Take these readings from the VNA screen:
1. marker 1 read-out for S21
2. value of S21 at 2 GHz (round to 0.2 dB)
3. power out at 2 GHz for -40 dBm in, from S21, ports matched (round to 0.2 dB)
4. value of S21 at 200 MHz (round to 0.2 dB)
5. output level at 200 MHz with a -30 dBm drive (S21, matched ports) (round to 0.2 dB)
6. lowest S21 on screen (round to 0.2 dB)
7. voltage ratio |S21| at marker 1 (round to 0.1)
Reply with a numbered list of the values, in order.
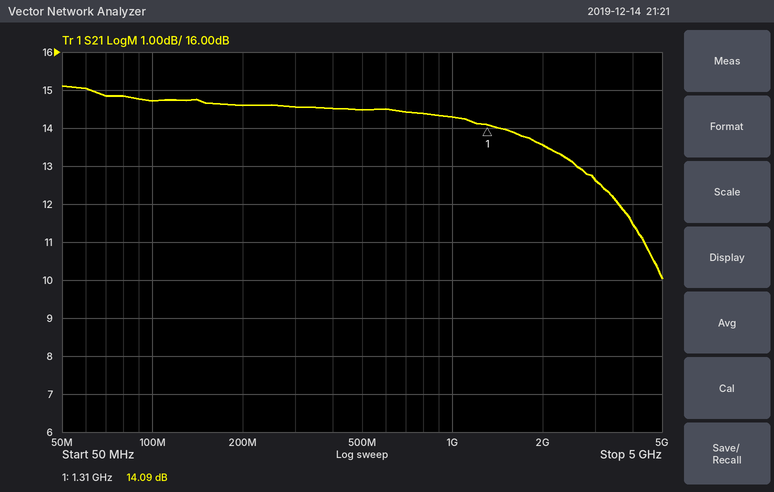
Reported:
1. 14.09 dB
2. 13.6 dB
3. -26.4 dBm
4. 14.6 dB
5. -15.4 dBm
6. 10.0 dB
7. 5.1
